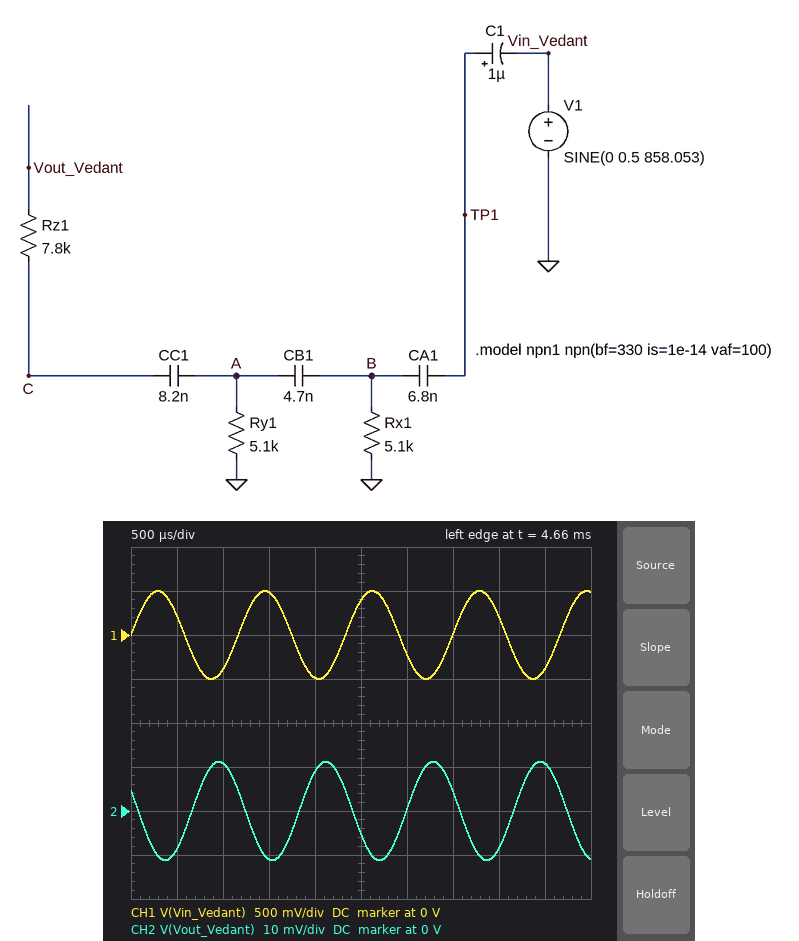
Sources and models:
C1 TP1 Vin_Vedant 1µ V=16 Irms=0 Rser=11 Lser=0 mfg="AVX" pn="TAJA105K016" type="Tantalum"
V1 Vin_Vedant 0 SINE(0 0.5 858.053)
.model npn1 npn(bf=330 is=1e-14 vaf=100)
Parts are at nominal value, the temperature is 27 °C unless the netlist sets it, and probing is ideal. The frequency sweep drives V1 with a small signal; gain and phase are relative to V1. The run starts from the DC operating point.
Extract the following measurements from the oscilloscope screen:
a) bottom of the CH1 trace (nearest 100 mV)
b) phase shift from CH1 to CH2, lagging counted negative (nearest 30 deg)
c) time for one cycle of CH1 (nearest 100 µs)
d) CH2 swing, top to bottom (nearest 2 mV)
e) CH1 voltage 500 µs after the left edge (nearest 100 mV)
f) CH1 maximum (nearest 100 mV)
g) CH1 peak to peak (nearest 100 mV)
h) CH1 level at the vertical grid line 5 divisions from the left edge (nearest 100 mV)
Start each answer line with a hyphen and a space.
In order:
- -500 mV
- 150 deg
- 1.2 ms
- 22 mV
- 200 mV
- 500 mV
- 1.0 V
- 400 mV
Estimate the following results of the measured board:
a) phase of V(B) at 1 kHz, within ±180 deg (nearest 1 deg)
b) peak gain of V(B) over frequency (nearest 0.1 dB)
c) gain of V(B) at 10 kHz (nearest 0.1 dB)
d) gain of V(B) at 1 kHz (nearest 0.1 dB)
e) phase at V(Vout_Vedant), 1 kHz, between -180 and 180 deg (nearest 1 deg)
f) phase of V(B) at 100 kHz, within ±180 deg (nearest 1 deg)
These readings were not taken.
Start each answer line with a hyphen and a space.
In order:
- 70 deg
- 0 dB
- -3.2 dB
- -14.0 dB
- 152 deg
- 5 deg
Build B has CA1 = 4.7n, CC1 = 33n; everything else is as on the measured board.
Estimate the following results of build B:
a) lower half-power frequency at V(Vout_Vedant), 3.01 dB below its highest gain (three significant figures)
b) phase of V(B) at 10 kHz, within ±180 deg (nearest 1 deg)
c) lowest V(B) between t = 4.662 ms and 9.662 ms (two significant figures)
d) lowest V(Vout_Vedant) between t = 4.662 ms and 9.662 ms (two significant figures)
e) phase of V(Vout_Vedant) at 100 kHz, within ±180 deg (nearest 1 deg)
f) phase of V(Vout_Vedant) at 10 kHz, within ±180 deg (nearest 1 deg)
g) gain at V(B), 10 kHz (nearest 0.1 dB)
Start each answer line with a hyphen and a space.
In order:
- 17.7 kHz
- 41 deg
- -61 mV
- -7.9 mV
- 11 deg
- 74 deg
- -4.8 dB
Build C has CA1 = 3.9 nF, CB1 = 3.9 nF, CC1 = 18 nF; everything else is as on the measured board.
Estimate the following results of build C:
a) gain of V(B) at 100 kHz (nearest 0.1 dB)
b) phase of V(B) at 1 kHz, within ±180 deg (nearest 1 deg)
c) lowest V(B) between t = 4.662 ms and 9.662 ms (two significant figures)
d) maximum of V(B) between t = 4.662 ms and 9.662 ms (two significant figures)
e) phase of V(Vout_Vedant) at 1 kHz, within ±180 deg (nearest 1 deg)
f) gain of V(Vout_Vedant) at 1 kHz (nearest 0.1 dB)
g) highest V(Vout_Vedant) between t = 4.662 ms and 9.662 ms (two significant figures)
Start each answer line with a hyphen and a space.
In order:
- -0.2 dB
- 76 deg
- -52 mV
- 52 mV
- 159 deg
- -36.6 dB
- 5.5 mV
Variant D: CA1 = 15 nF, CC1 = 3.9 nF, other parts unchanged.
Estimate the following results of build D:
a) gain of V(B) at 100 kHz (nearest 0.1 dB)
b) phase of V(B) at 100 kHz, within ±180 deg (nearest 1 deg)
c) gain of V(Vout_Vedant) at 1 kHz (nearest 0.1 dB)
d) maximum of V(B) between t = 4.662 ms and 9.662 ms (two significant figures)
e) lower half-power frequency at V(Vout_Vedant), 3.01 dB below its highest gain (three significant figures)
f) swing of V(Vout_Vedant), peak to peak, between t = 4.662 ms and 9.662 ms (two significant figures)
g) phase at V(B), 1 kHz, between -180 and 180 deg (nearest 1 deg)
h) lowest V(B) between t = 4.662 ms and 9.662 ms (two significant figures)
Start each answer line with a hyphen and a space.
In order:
- -0.1 dB
- 2 deg
- -24.6 dB
- 180 mV
- 9.57 kHz
- 45 mV
- 59 deg
- -180 mV
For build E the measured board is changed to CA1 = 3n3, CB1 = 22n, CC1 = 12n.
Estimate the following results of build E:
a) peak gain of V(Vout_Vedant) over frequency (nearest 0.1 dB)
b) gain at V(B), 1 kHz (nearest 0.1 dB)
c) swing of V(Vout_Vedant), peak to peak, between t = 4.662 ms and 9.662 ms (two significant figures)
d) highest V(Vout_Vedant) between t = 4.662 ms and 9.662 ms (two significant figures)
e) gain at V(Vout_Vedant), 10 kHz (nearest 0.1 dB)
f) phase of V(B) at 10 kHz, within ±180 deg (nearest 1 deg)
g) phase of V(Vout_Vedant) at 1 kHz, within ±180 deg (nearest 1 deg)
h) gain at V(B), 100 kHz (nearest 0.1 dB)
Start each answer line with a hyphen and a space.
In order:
- 0 dB
- -22.8 dB
- 34 mV
- 17 mV
- -6.9 dB
- 59 deg
- 121 deg
- -0.2 dB
